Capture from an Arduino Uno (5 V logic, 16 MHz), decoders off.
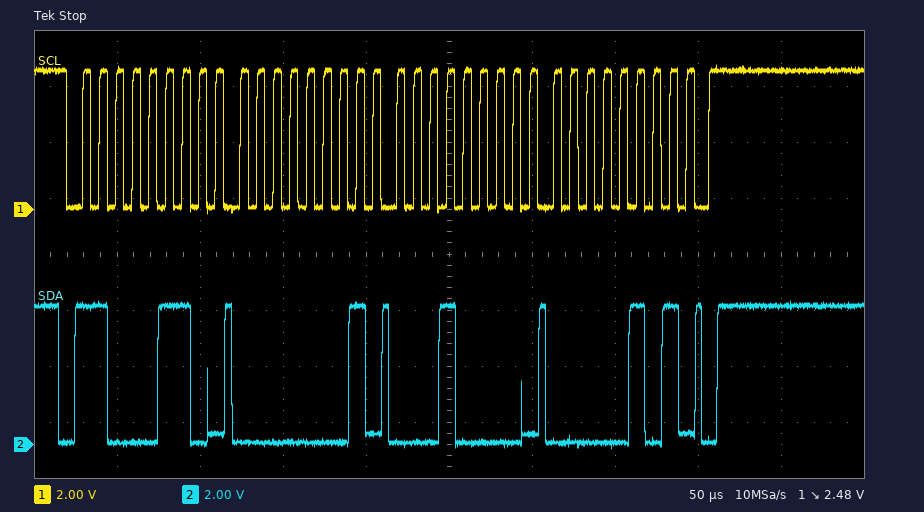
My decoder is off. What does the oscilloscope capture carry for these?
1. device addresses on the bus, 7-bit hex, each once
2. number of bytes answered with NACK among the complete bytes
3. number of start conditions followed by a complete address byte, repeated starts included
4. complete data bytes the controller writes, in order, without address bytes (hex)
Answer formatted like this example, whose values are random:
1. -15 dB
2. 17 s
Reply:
1. 0x63
2. 0
3. 1
4. 01 10 05
